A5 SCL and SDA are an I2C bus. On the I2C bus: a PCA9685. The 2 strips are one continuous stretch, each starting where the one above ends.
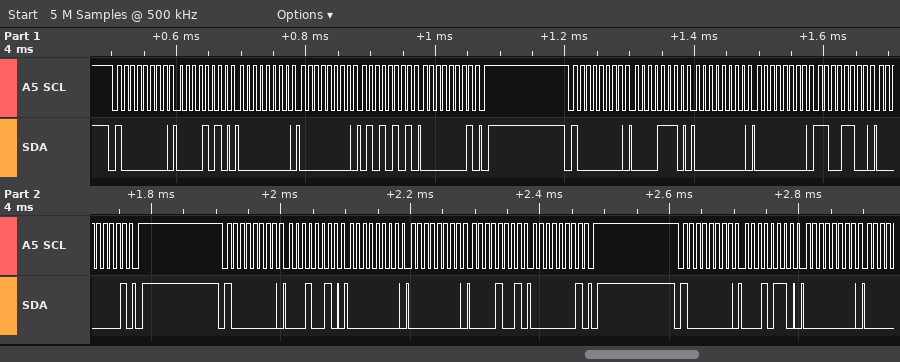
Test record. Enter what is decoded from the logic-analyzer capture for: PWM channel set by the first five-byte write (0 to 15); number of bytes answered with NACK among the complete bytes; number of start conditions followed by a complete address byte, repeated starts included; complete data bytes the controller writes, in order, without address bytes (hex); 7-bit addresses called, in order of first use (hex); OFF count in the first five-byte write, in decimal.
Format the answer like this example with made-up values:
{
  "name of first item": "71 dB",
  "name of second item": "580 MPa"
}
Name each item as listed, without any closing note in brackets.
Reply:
{
  "PWM channel set by the first five-byte write": "1",
  "number of bytes answered with NACK among the complete bytes": "0",
  "number of start conditions followed by a complete address byte, repeated starts included": "4",
  "complete data bytes the controller writes, in order, without address bytes": "0A 00 00 55 01 0E 00 00 CC 01 12 00 00 09 01 16 00",
  "7-bit addresses called, in order of first use": "0x40",
  "OFF count in the first five-byte write, in decimal": "341"
}
